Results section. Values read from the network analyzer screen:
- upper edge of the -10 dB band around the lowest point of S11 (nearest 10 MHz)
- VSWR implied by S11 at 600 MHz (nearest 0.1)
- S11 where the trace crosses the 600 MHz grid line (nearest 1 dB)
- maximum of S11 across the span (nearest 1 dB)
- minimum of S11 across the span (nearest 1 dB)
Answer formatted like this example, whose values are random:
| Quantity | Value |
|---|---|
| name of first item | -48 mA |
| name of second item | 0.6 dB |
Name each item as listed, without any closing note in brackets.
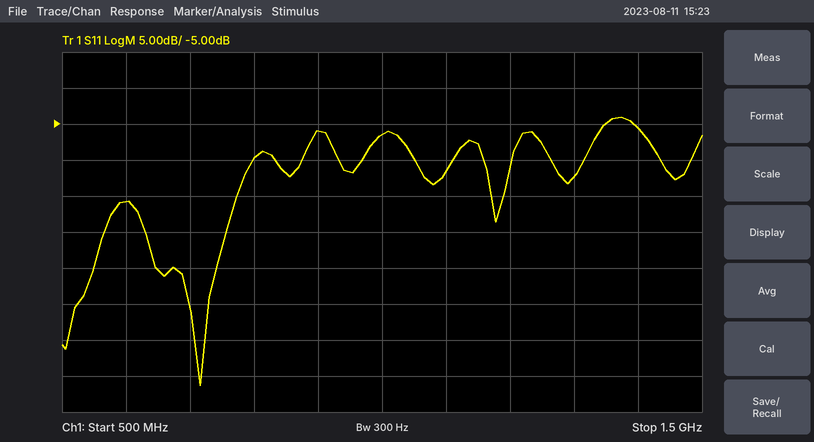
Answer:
| Quantity | Value |
|---|---|
| upper edge of the -10 dB band around the lowest point of S11 | 800 MHz |
| VSWR implied by S11 at 600 MHz | 1.4 |
| S11 where the trace crosses the 600 MHz grid line | -16 dB |
| maximum of S11 across the span | -4 dB |
| minimum of S11 across the span | -41 dB |
